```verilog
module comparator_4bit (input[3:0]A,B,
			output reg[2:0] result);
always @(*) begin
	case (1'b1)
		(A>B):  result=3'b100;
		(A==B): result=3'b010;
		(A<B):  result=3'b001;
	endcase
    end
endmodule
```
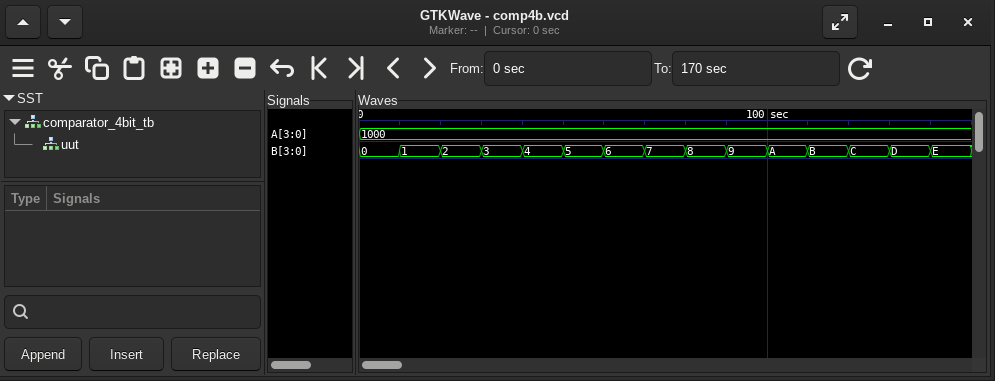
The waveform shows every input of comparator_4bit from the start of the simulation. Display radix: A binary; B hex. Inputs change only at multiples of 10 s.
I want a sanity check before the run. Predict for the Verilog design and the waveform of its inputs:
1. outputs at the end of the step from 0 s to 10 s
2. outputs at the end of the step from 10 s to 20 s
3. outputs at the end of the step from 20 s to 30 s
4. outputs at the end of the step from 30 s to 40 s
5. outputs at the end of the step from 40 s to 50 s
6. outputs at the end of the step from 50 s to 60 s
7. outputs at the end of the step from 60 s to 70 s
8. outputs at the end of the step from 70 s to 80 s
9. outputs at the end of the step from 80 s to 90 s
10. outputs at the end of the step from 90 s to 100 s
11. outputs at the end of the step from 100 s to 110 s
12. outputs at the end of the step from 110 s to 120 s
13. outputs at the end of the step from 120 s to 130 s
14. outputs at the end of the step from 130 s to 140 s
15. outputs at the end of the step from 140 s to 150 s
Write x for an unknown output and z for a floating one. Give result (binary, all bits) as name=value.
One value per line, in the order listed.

result=100
result=100
result=100
result=100
result=100
result=100
result=100
result=100
result=010
result=001
result=001
result=001
result=001
result=001
result=001
